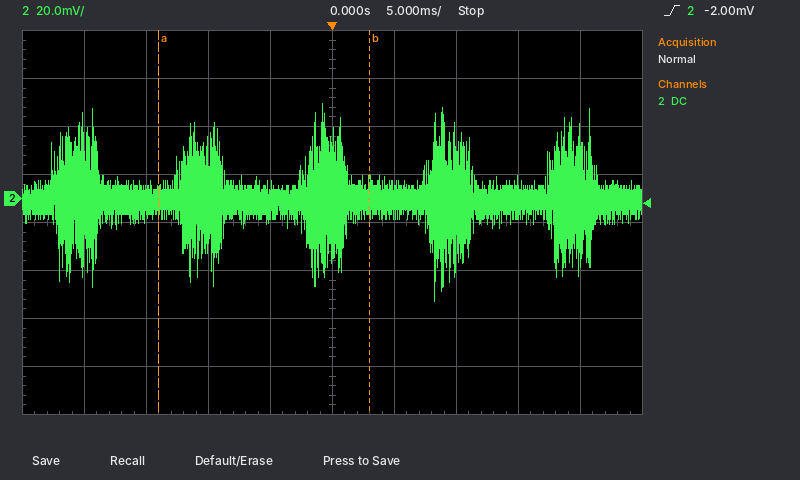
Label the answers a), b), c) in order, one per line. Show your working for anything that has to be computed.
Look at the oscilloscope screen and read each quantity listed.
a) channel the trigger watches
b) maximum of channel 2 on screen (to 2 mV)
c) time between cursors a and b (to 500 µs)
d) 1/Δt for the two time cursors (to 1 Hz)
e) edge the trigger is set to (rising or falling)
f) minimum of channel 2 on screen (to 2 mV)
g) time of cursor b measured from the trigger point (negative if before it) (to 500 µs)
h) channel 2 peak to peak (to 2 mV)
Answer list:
a) channel 2
b) 40 mV
c) 17.0 ms
d) 1 / 17.0 ms ≈ 59 Hz
e) rising
f) -42 mV
g) +3.0 ms
h) 40 mV − (-42 mV) = 82 mV
